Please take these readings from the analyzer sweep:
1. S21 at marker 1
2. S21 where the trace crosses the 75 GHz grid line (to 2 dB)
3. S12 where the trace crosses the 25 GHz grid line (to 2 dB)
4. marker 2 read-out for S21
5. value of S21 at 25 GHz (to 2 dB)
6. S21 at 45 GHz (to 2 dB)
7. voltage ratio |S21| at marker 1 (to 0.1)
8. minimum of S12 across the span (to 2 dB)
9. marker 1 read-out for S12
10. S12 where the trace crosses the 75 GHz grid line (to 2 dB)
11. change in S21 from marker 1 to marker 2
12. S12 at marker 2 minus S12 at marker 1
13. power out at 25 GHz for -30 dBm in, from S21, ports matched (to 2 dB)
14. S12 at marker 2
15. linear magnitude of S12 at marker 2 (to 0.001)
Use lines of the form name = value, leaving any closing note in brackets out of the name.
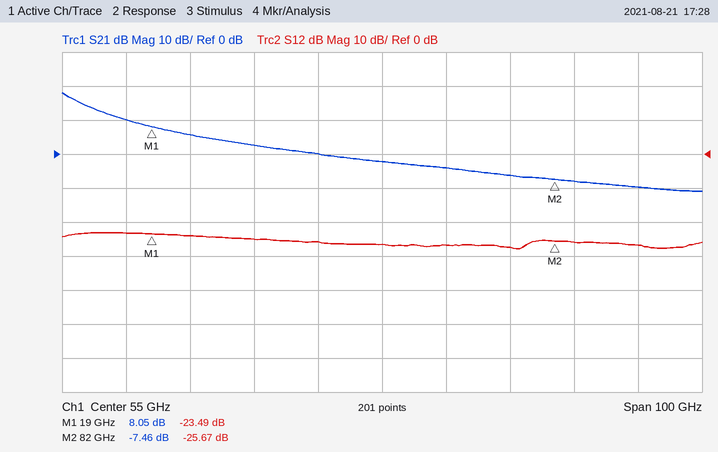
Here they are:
S21 at marker 1 = 8.05 dB
S21 where the trace crosses the 75 GHz grid line = -6 dB
S12 where the trace crosses the 25 GHz grid line = -24 dB
marker 2 read-out for S21 = -7.46 dB
value of S21 at 25 GHz = 6 dB
S21 at 45 GHz = 0 dB
voltage ratio |S21| at marker 1 = 2.5
minimum of S12 across the span = -28 dB
marker 1 read-out for S12 = -23.49 dB
S12 where the trace crosses the 75 GHz grid line = -28 dB
change in S21 from marker 1 to marker 2 = -15.51 dB
S12 at marker 2 minus S12 at marker 1 = -2.18 dB
power out at 25 GHz for -30 dBm in, from S21, ports matched = -24 dBm
S12 at marker 2 = -25.67 dB
linear magnitude of S12 at marker 2 = 0.052
